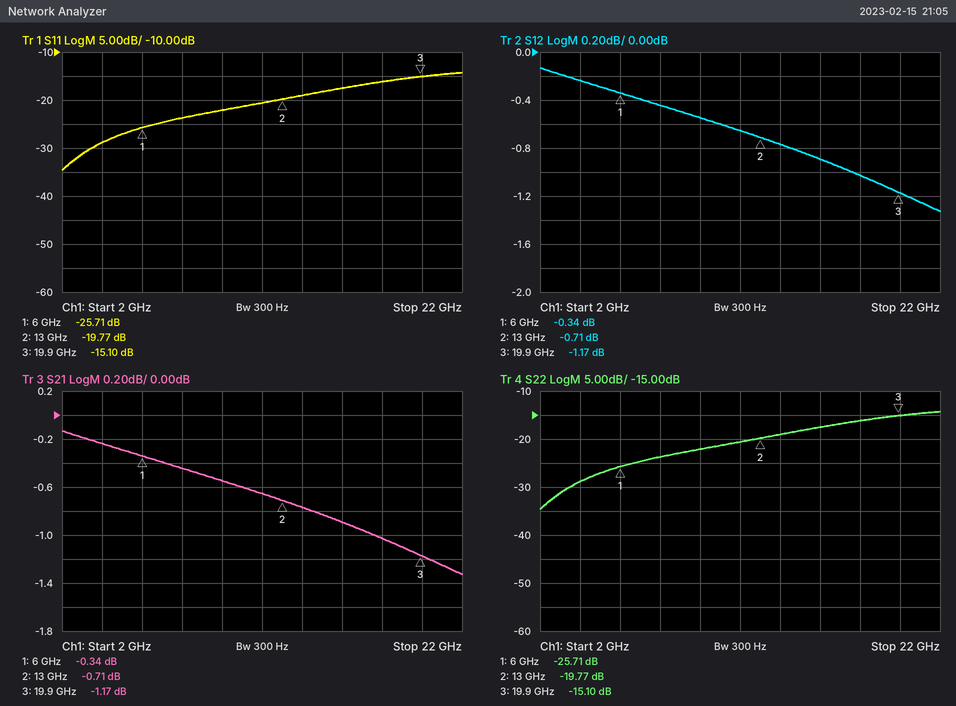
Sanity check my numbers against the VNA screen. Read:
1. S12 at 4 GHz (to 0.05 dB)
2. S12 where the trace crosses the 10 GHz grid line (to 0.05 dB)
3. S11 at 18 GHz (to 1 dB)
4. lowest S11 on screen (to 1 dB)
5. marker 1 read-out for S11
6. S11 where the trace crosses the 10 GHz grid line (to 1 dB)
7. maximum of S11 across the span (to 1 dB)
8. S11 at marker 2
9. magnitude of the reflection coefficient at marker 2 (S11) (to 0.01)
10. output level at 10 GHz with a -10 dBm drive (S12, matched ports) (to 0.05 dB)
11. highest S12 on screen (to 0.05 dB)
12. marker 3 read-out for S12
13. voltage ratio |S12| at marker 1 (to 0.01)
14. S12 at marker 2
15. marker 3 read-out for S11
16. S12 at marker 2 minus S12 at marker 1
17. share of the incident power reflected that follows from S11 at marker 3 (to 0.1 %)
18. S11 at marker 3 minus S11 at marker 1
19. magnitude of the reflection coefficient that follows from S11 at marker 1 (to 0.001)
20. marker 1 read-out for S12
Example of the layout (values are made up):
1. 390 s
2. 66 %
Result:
1. -0.25 dB
2. -0.55 dB
3. -16 dB
4. -35 dB
5. -25.71 dB
6. -22 dB
7. -14 dB
8. -19.77 dB
9. 0.10
10. -10.55 dBm
11. -0.15 dB
12. -1.17 dB
13. 0.96
14. -0.71 dB
15. -15.10 dB
16. -0.37 dB
17. 3.1 %
18. 10.61 dB
19. 0.052
20. -0.34 dB
